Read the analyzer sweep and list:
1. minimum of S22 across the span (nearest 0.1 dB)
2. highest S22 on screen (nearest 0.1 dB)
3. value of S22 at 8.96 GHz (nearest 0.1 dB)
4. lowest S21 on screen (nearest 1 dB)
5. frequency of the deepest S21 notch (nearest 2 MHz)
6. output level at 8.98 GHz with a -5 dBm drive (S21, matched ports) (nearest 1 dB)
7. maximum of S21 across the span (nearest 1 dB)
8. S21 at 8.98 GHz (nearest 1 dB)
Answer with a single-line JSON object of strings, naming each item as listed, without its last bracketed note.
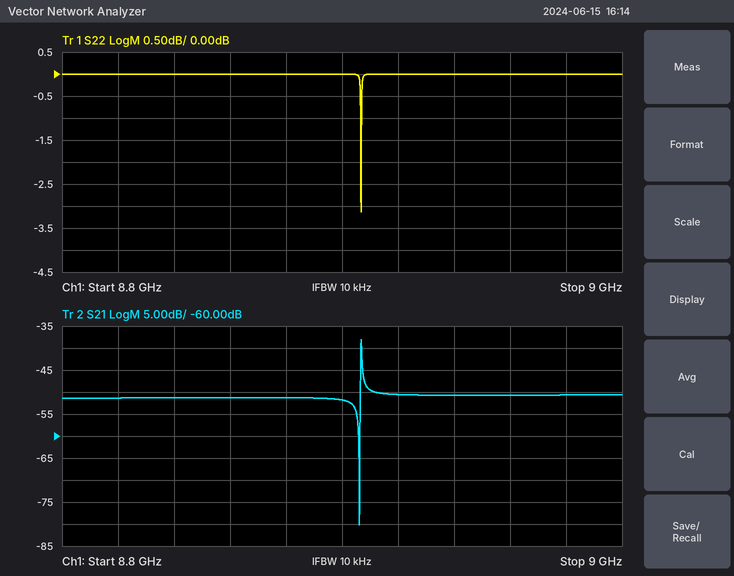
{"minimum of S22 across the span": "-3.1 dB", "highest S22 on screen": "0.0 dB", "value of S22 at 8.96 GHz": "0.0 dB", "lowest S21 on screen": "-80 dB", "frequency of the deepest S21 notch": "8.906 GHz", "output level at 8.98 GHz with a -5 dBm drive (S21, matched ports)": "-56 dBm", "maximum of S21 across the span": "-38 dB", "S21 at 8.98 GHz": "-51 dB"}
